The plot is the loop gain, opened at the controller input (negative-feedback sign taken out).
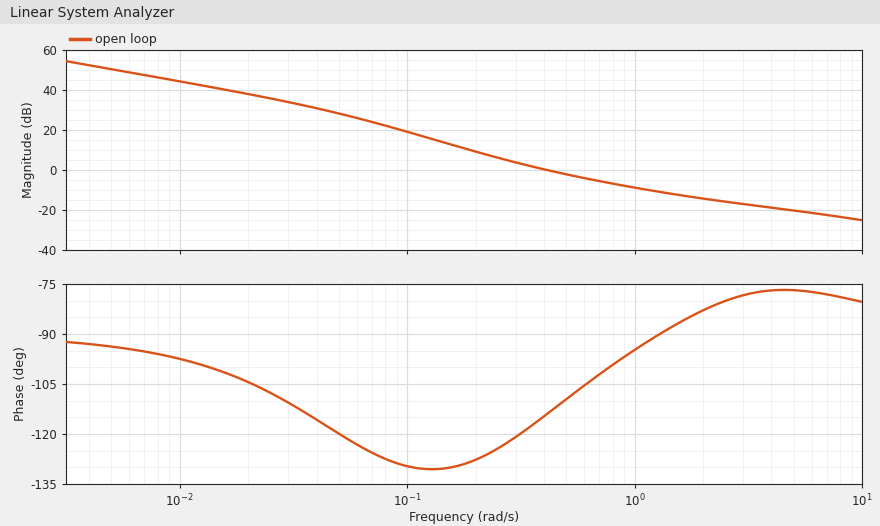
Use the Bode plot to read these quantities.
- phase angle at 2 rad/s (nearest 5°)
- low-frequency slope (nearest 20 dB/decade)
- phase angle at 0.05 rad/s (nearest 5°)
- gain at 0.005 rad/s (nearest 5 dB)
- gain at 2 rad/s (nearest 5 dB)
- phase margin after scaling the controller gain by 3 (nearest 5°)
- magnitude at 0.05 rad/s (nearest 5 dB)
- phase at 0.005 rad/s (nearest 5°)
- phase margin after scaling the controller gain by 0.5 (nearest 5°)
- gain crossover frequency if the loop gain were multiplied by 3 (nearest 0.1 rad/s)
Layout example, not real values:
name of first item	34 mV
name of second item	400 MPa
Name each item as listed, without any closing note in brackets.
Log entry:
phase angle at 2 rad/s	-85°
low-frequency slope	-20 dB/decade
phase angle at 0.05 rad/s	-120°
gain at 0.005 rad/s	50 dB
gain at 2 rad/s	-15 dB
phase margin after scaling the controller gain by 3	85°
magnitude at 0.05 rad/s	30 dB
phase at 0.005 rad/s	-95°
phase margin after scaling the controller gain by 0.5	55°
gain crossover frequency if the loop gain were multiplied by 3	1.1 rad/s
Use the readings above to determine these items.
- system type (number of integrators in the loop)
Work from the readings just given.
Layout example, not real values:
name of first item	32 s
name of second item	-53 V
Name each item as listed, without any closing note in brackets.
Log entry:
system type	1
